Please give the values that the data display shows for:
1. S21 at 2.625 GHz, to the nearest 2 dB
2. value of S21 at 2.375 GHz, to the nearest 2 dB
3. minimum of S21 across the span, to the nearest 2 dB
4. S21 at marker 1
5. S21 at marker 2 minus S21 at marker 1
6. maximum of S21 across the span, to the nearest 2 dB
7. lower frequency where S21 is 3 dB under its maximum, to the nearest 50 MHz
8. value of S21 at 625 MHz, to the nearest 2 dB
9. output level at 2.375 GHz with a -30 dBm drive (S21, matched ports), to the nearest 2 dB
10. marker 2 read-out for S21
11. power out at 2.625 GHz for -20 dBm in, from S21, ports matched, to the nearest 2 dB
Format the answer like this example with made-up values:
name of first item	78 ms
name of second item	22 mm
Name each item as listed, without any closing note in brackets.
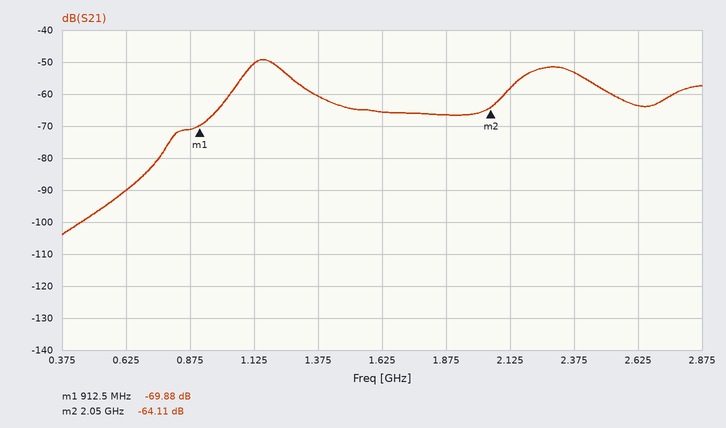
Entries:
S21 at 2.625 GHz, to the nearest 2 dB	-64 dB
value of S21 at 2.375 GHz, to the nearest 2 dB	-54 dB
minimum of S21 across the span, to the nearest 2 dB	-104 dB
S21 at marker 1	-69.88 dB
S21 at marker 2 minus S21 at marker 1	5.77 dB
maximum of S21 across the span, to the nearest 2 dB	-50 dB
lower frequency where S21 is 3 dB under its maximum, to the nearest 50 MHz	1.10 GHz
value of S21 at 625 MHz, to the nearest 2 dB	-90 dB
output level at 2.375 GHz with a -30 dBm drive (S21, matched ports), to the nearest 2 dB	-84 dBm
marker 2 read-out for S21	-64.11 dB
power out at 2.625 GHz for -20 dBm in, from S21, ports matched, to the nearest 2 dB	-84 dBm
